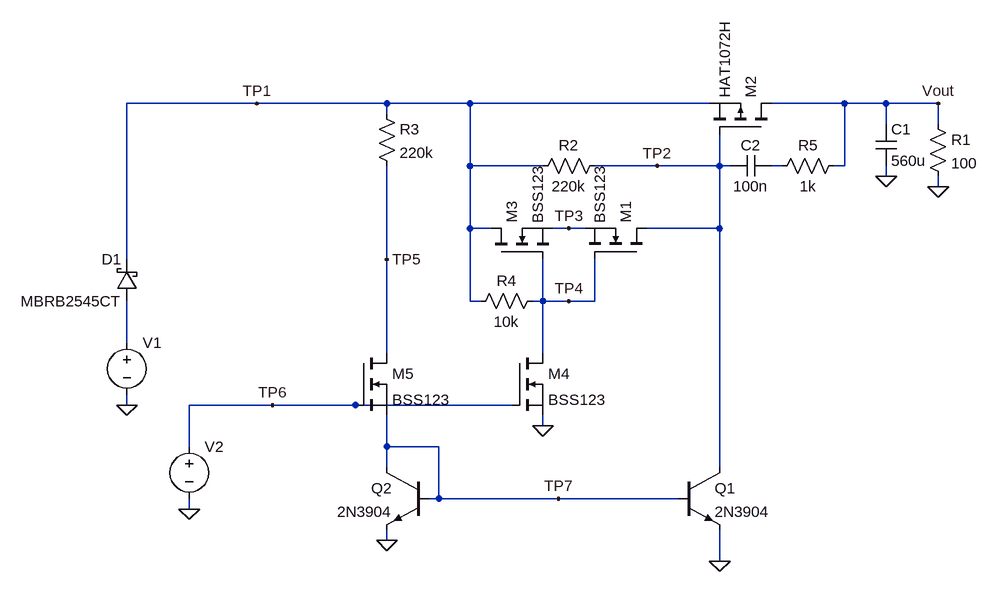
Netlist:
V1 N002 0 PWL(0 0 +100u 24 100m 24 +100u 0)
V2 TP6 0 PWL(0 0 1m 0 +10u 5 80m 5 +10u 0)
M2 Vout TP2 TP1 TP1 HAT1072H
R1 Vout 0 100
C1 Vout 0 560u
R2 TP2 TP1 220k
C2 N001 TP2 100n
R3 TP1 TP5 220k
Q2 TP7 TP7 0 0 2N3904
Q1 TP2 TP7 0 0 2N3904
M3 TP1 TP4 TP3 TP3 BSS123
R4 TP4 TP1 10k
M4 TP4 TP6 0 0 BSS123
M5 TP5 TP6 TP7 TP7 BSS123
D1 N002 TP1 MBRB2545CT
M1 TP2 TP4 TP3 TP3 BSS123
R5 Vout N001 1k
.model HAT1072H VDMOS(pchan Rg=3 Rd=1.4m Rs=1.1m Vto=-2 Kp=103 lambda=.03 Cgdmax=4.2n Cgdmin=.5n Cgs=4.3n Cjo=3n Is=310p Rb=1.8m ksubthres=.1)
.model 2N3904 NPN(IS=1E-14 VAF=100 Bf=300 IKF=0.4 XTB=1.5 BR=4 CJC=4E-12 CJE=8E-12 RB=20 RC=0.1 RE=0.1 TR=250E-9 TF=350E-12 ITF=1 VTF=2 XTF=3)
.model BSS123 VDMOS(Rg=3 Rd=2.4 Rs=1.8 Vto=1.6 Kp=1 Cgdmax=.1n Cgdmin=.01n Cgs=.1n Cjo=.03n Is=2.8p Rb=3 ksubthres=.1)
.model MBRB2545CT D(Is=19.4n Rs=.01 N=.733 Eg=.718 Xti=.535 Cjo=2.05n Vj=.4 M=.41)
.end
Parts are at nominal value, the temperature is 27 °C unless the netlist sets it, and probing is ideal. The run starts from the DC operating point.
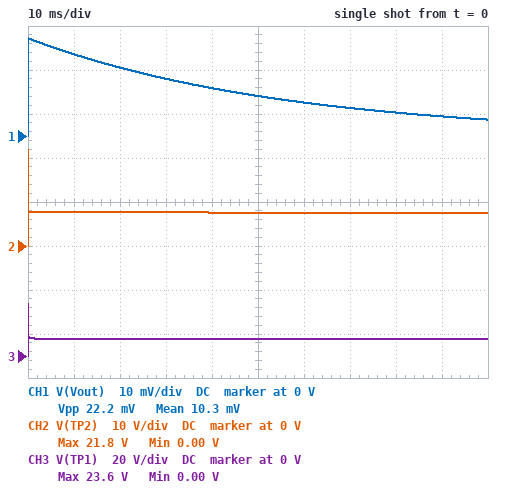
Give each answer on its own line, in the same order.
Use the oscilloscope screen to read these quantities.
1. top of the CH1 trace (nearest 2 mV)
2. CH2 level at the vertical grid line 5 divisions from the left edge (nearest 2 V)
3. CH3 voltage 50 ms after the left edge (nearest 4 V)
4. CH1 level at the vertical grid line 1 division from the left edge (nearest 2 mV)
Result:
22 mV
8 V
8 V
18 mV
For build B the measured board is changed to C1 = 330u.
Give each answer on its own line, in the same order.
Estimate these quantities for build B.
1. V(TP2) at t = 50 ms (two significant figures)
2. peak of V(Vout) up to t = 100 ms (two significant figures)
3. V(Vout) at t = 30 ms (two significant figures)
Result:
7.6 V
37 mV
15 mV
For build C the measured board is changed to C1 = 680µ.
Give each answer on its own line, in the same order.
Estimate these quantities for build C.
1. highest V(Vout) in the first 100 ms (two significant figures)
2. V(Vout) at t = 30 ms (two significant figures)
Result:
18 mV
12 mV
